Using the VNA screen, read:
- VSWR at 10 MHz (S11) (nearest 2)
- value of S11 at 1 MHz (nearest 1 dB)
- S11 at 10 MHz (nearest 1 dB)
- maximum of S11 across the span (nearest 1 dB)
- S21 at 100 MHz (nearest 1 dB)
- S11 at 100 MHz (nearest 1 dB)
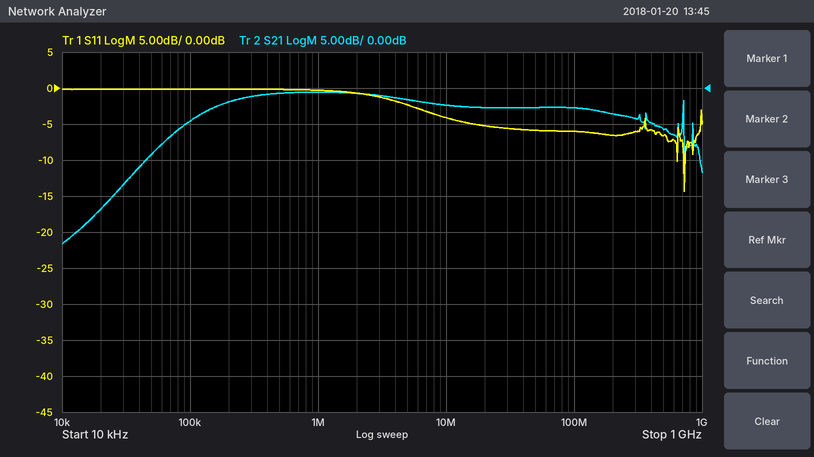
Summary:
4
0 dB
-4 dB
0 dB
-3 dB
-6 dB
